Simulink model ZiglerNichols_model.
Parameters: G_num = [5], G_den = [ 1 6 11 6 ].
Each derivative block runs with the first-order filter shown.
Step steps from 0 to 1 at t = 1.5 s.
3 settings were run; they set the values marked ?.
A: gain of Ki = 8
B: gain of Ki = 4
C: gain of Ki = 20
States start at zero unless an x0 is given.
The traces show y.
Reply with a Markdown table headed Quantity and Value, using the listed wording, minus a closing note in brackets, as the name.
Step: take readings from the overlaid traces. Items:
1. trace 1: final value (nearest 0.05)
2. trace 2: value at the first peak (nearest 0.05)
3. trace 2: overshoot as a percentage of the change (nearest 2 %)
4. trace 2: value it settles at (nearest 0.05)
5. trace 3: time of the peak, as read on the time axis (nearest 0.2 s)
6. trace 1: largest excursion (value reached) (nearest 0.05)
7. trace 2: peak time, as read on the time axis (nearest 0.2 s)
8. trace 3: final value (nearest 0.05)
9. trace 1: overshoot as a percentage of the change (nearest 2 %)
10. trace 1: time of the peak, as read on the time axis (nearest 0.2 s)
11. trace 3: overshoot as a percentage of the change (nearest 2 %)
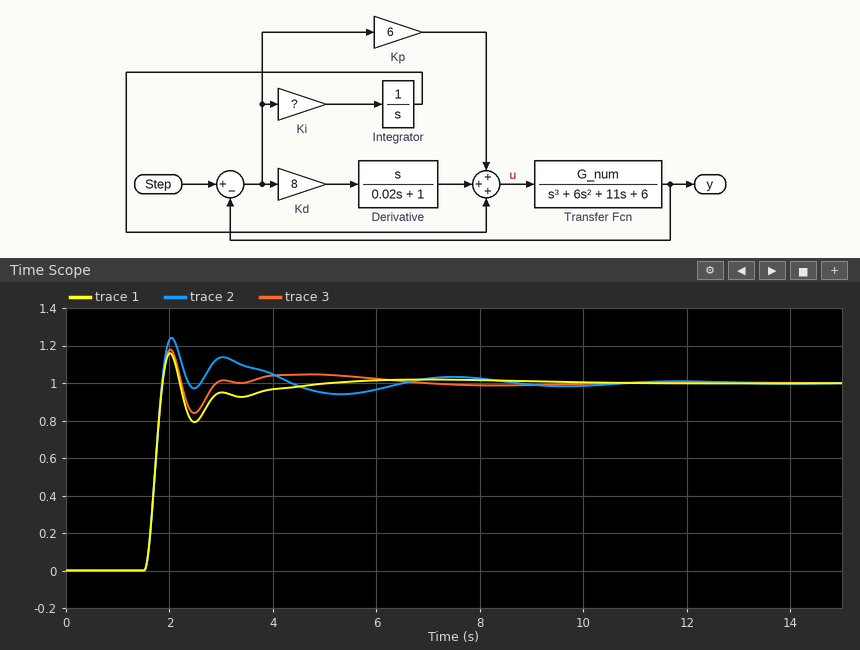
| Quantity | Value |
|---|---|
| trace 1: final value | 1.00 |
| trace 2: value at the first peak | 1.25 |
| trace 2: overshoot as a percentage of the change | 24 % |
| trace 2: value it settles at | 1.00 |
| trace 3: time of the peak, as read on the time axis | 2.0 s |
| trace 1: largest excursion (value reached) | 1.15 |
| trace 2: peak time, as read on the time axis | 2.0 s |
| trace 3: final value | 1.00 |
| trace 1: overshoot as a percentage of the change | 16 % |
| trace 1: time of the peak, as read on the time axis | 2.0 s |
| trace 3: overshoot as a percentage of the change | 18 % |
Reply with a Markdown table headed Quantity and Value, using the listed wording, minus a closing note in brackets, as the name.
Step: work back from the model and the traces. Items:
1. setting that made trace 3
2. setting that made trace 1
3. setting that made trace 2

| Quantity | Value |
|---|---|
| setting that made trace 3 | A |
| setting that made trace 1 | B |
| setting that made trace 2 | C |
